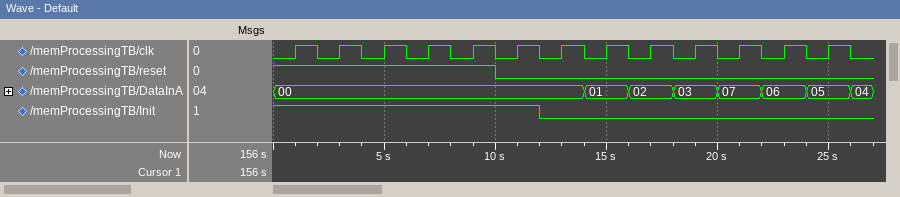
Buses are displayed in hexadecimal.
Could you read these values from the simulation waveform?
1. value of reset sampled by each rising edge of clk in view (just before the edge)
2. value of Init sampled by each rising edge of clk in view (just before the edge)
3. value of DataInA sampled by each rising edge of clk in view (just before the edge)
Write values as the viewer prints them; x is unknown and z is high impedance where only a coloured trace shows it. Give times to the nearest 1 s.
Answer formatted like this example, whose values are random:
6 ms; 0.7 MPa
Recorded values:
1 1 1 1 1 0 0 0 0 0 0 0 0; 1 1 1 1 1 1 0 0 0 0 0 0 0; 00, 00, 00, 00, 00, 00, 00, 01, 02, 03, 07, 06, 05
